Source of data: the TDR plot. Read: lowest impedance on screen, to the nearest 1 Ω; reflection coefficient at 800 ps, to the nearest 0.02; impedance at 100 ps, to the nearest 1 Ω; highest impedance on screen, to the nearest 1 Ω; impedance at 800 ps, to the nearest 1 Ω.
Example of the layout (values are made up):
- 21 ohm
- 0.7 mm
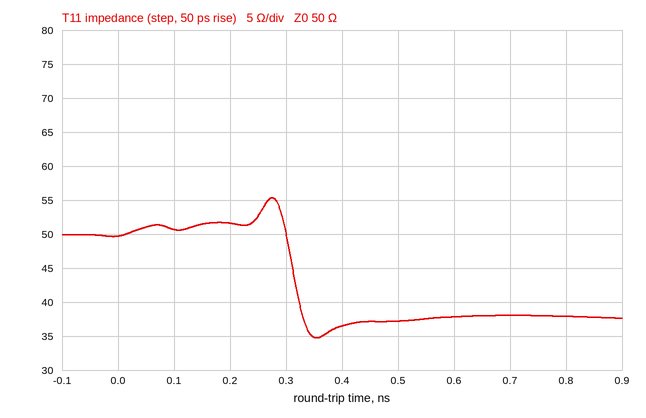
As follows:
- 35 Ω
- -0.14
- 51 Ω
- 55 Ω
- 38 Ω
